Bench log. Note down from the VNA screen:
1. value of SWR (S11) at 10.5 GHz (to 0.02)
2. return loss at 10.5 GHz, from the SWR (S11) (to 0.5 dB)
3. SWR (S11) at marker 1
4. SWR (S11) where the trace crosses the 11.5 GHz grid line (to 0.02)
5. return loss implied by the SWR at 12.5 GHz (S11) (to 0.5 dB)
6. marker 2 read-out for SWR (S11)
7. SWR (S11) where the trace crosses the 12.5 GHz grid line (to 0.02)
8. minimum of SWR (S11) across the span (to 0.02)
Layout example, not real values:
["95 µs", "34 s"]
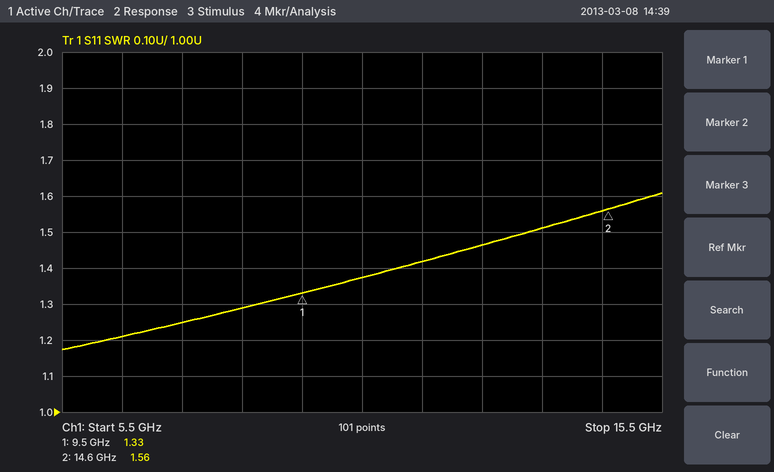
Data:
["1.38", "16.0 dB", "1.33", "1.42", "14.5 dB", "1.56", "1.46", "1.18"]
